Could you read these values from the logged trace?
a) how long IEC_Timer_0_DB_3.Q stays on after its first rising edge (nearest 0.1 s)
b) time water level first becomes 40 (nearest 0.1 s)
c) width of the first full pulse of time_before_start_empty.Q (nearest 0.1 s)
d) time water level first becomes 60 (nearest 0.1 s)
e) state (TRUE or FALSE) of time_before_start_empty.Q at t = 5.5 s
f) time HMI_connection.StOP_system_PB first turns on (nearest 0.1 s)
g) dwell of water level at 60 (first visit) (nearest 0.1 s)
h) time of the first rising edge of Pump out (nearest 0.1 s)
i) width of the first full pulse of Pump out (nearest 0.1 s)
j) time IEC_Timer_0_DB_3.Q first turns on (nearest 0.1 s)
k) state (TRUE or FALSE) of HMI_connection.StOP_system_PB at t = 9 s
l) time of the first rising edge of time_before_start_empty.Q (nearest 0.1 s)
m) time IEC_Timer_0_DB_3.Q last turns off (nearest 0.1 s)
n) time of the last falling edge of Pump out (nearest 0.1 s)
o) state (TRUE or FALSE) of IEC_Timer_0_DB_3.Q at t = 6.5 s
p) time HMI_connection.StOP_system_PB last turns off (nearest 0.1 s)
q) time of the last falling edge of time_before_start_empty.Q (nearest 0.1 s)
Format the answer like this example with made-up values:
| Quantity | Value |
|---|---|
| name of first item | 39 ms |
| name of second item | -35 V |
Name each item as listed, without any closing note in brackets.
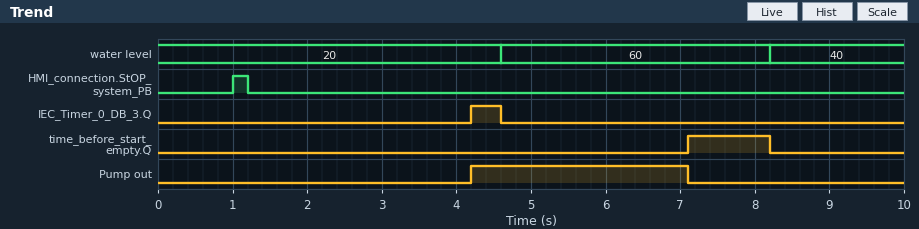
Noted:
| Quantity | Value |
|---|---|
| how long IEC_Timer_0_DB_3.Q stays on after its first rising edge | 0.4 s |
| time water level first becomes 40 | 8.2 s |
| width of the first full pulse of time_before_start_empty.Q | 1.1 s |
| time water level first becomes 60 | 4.6 s |
| state (TRUE or FALSE) of time_before_start_empty.Q at t = 5.5 s | FALSE |
| time HMI_connection.StOP_system_PB first turns on | 1.0 s |
| dwell of water level at 60 (first visit) | 3.6 s |
| time of the first rising edge of Pump out | 4.2 s |
| width of the first full pulse of Pump out | 2.9 s |
| time IEC_Timer_0_DB_3.Q first turns on | 4.2 s |
| state (TRUE or FALSE) of HMI_connection.StOP_system_PB at t = 9 s | FALSE |
| time of the first rising edge of time_before_start_empty.Q | 7.1 s |
| time IEC_Timer_0_DB_3.Q last turns off | 4.6 s |
| time of the last falling edge of Pump out | 7.1 s |
| state (TRUE or FALSE) of IEC_Timer_0_DB_3.Q at t = 6.5 s | FALSE |
| time HMI_connection.StOP_system_PB last turns off | 1.2 s |
| time of the last falling edge of time_before_start_empty.Q | 8.2 s |
